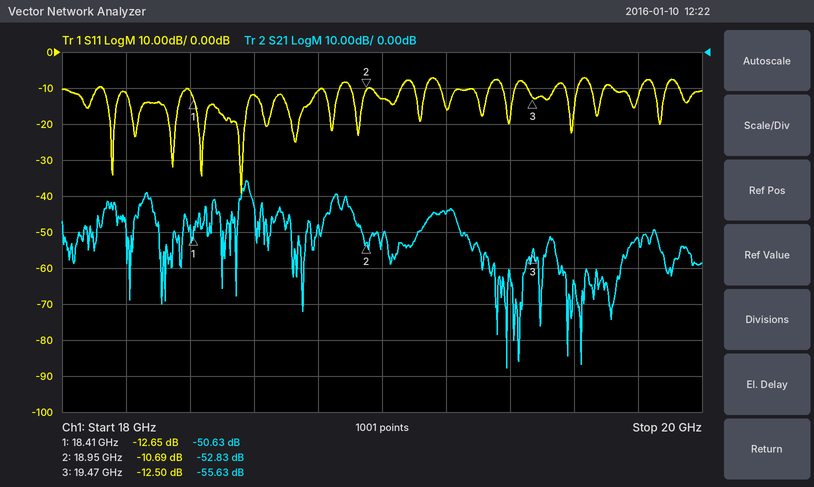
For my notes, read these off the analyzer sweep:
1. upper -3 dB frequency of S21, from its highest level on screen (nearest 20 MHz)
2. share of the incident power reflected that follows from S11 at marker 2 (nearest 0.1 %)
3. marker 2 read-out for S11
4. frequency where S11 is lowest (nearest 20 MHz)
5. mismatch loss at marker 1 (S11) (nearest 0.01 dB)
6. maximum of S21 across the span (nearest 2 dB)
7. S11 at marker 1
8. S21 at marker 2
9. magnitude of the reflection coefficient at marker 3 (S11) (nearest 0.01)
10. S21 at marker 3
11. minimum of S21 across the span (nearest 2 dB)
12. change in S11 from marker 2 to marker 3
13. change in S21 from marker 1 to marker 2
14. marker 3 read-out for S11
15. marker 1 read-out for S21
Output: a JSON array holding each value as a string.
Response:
["18.58 GHz", "8.5 %", "-10.69 dB", "18.56 GHz", "0.24 dB", "-36 dB", "-12.65 dB", "-52.83 dB", "0.24", "-55.63 dB", "-88 dB", "-1.81 dB", "-2.20 dB", "-12.50 dB", "-50.63 dB"]
